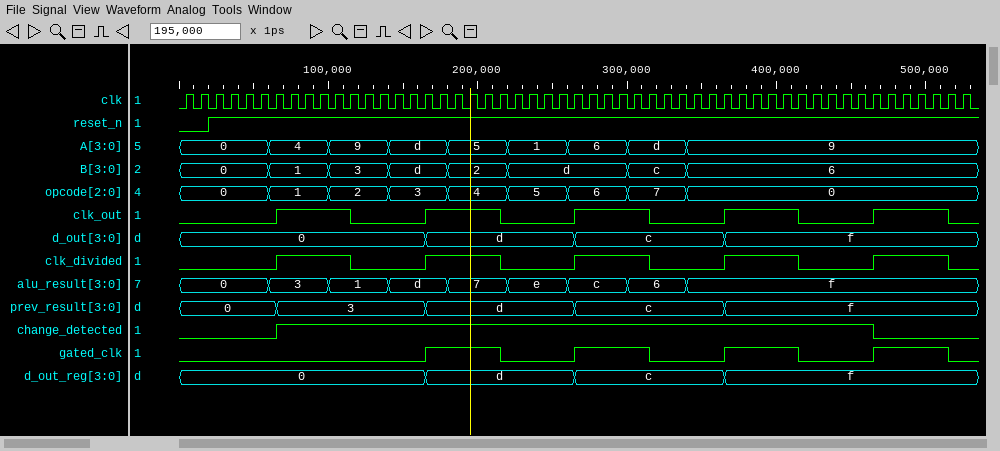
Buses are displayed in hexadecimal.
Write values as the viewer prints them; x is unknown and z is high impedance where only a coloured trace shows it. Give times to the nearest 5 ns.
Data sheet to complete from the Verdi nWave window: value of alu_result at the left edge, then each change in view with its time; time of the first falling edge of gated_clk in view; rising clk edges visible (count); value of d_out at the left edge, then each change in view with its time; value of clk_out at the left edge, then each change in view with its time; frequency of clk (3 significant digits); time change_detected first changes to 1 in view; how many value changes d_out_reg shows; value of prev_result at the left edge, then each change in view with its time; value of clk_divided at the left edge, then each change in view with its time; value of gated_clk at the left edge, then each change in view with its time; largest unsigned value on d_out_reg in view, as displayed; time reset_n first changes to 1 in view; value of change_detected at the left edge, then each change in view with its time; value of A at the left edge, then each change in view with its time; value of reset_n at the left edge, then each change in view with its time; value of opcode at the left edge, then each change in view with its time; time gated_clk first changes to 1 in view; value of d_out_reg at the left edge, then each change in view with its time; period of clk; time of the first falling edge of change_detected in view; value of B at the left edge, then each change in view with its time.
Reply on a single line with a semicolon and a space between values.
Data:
0, 3 at 60 ns, 1 at 100 ns, d at 140 ns, 7 at 180 ns, e at 220 ns, c at 260 ns, 6 at 300 ns, f at 340 ns; 215 ns; 53; 0, d at 165 ns, c at 265 ns, f at 365 ns; 0, 1 at 65 ns, 0 at 115 ns, 1 at 165 ns, 0 at 215 ns, 1 at 265 ns, 0 at 315 ns, 1 at 365 ns, 0 at 415 ns, 1 at 465 ns, 0 at 515 ns; 100 MHz; 65 ns; 3; 0, 3 at 65 ns, d at 165 ns, c at 265 ns, f at 365 ns; 0, 1 at 65 ns, 0 at 115 ns, 1 at 165 ns, 0 at 215 ns, 1 at 265 ns, 0 at 315 ns, 1 at 365 ns, 0 at 415 ns, 1 at 465 ns, 0 at 515 ns; 0, 1 at 165 ns, 0 at 215 ns, 1 at 265 ns, 0 at 315 ns, 1 at 365 ns, 0 at 415 ns, 1 at 465 ns, 0 at 515 ns; f; 20 ns; 0, 1 at 65 ns, 0 at 465 ns; 0, 4 at 60 ns, 9 at 100 ns, d at 140 ns, 5 at 180 ns, 1 at 220 ns, 6 at 260 ns, d at 300 ns, 9 at 340 ns; 0, 1 at 20 ns; 0, 1 at 60 ns, 2 at 100 ns, 3 at 140 ns, 4 at 180 ns, 5 at 220 ns, 6 at 260 ns, 7 at 300 ns, 0 at 340 ns; 165 ns; 0, d at 165 ns, c at 265 ns, f at 365 ns; 10 ns; 465 ns; 0, 1 at 60 ns, 3 at 100 ns, d at 140 ns, 2 at 180 ns, d at 220 ns, c at 300 ns, 6 at 340 ns
